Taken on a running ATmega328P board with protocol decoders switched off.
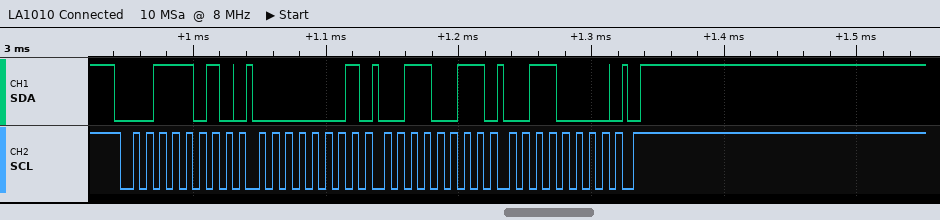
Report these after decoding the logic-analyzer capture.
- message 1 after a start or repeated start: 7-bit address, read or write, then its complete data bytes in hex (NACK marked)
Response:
0x1D write: 01 33 30
